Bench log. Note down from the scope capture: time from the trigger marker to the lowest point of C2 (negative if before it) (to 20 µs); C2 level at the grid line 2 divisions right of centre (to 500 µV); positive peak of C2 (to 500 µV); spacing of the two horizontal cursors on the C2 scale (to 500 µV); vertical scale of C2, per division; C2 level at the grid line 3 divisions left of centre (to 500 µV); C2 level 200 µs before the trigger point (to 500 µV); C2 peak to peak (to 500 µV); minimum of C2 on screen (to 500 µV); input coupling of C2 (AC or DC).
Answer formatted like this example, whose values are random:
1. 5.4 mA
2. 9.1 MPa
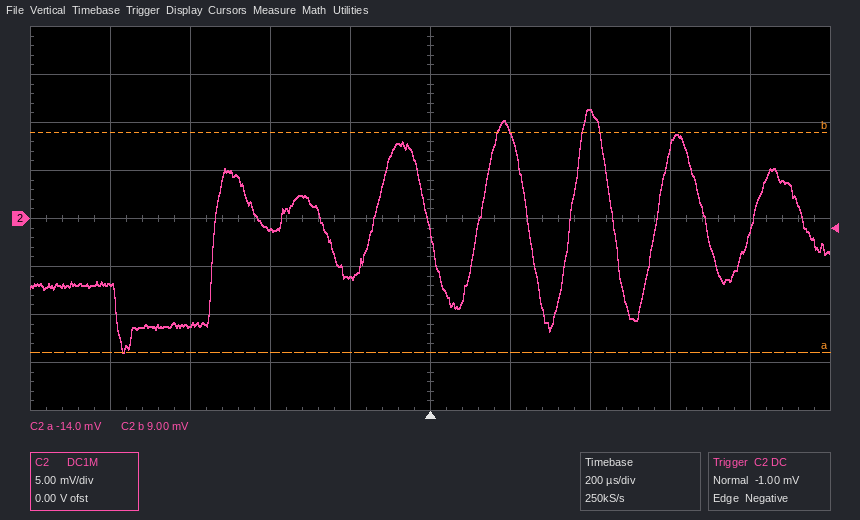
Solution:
1. -760 µs
2. 11.0 mV
3. 11.5 mV
4. 23.0 mV
5. 5 mV
6. -11.0 mV
7. -6.0 mV
8. 25.5 mV
9. -14.0 mV
10. DC
